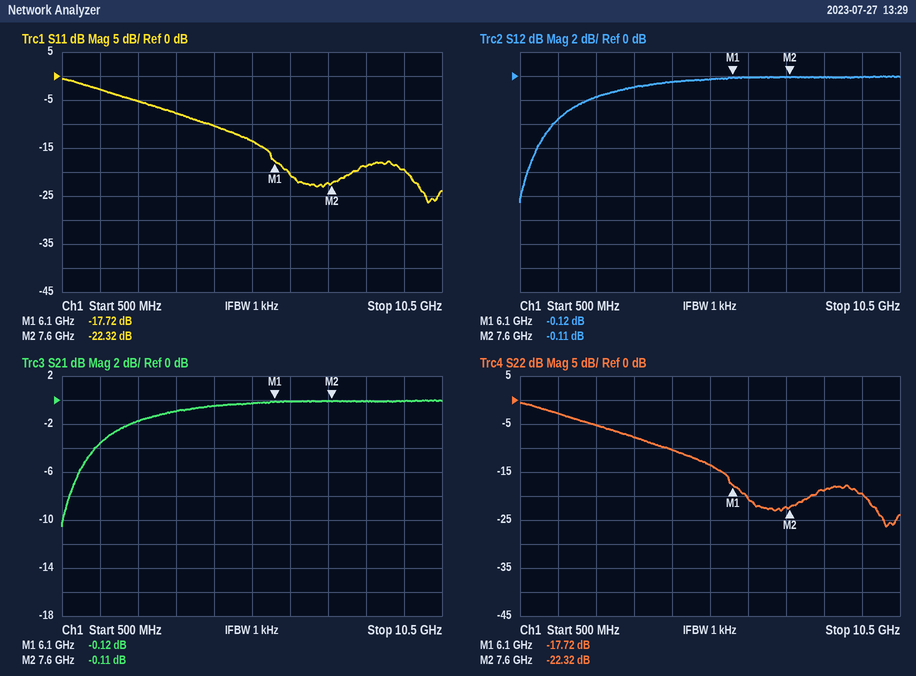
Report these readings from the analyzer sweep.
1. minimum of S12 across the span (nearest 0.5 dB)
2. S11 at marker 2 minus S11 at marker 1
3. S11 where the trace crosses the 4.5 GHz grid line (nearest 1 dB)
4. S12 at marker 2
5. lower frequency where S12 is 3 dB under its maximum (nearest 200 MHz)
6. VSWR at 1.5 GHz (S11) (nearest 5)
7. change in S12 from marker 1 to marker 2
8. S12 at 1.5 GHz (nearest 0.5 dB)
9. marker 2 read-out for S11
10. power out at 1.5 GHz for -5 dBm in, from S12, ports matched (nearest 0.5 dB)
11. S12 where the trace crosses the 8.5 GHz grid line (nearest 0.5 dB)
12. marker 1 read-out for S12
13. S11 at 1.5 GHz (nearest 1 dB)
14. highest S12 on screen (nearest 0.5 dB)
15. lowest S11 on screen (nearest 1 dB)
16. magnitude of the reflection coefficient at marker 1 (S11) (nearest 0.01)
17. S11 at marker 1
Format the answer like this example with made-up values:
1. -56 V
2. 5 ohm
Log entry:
1. -10.5 dB
2. -4.60 dB
3. -10 dB
4. -0.11 dB
5. 1.8 GHz
6. 5
7. 0.01 dB
8. -3.5 dB
9. -22.32 dB
10. -8.5 dBm
11. 0.0 dB
12. -0.12 dB
13. -3 dB
14. 0.0 dB
15. -26 dB
16. 0.13
17. -17.72 dB
